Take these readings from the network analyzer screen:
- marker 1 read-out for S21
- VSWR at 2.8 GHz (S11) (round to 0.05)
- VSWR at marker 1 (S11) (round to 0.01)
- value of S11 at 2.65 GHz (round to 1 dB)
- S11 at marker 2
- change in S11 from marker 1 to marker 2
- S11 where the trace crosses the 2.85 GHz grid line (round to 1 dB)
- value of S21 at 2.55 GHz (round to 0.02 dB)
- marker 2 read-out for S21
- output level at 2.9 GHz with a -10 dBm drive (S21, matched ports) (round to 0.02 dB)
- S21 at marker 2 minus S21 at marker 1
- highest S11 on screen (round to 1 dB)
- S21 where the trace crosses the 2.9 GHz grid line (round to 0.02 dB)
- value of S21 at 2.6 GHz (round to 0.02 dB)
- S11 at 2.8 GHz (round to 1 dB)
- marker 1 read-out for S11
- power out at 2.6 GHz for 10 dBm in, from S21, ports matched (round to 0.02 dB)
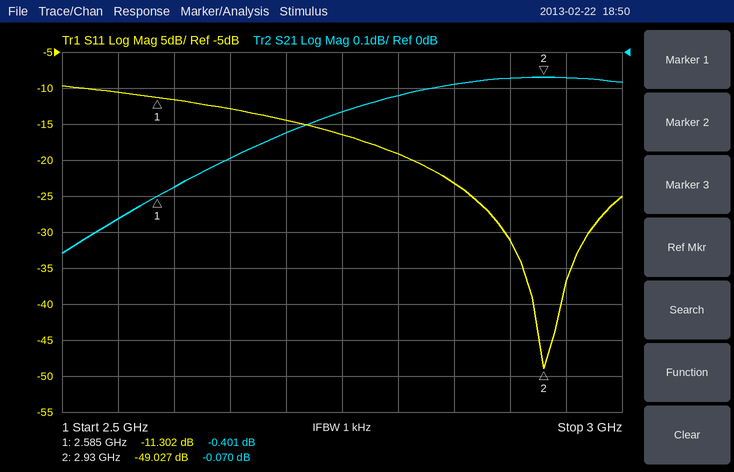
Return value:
-0.401 dB
1.25
1.75
-13 dB
-49.027 dB
-37.725 dB
-23 dB
-0.46 dB
-0.070 dB
-10.08 dBm
0.331 dB
-10 dB
-0.08 dB
-0.38 dB
-19 dB
-11.302 dB
9.62 dBm
